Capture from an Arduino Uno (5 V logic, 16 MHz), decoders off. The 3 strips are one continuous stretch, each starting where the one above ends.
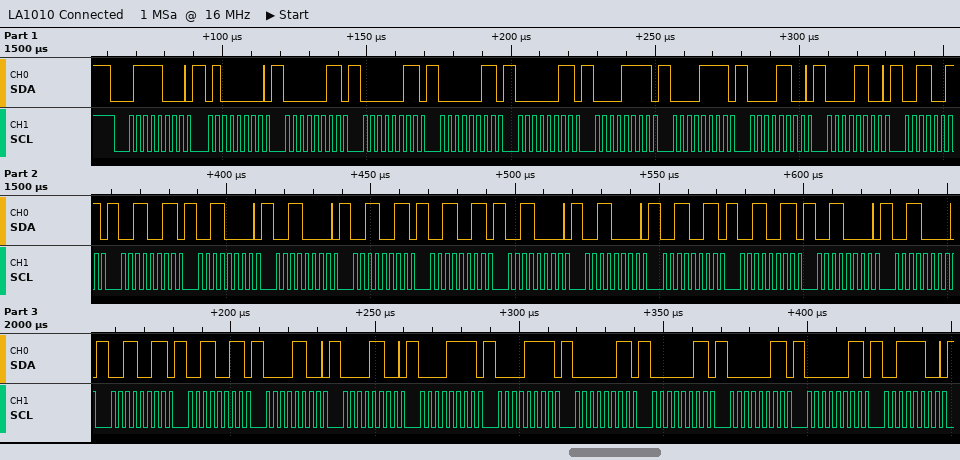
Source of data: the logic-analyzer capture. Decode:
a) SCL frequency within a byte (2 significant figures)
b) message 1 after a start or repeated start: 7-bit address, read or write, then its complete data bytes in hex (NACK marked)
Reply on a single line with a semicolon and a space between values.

400 kHz; 0x3C write: 40 03 03 03 03 0F 0F 0C 0C 33 33 30 30 33 33 30 30 33 33 30 30 33 33 0C 0C 0F 0F 03 03 03 03 3C
